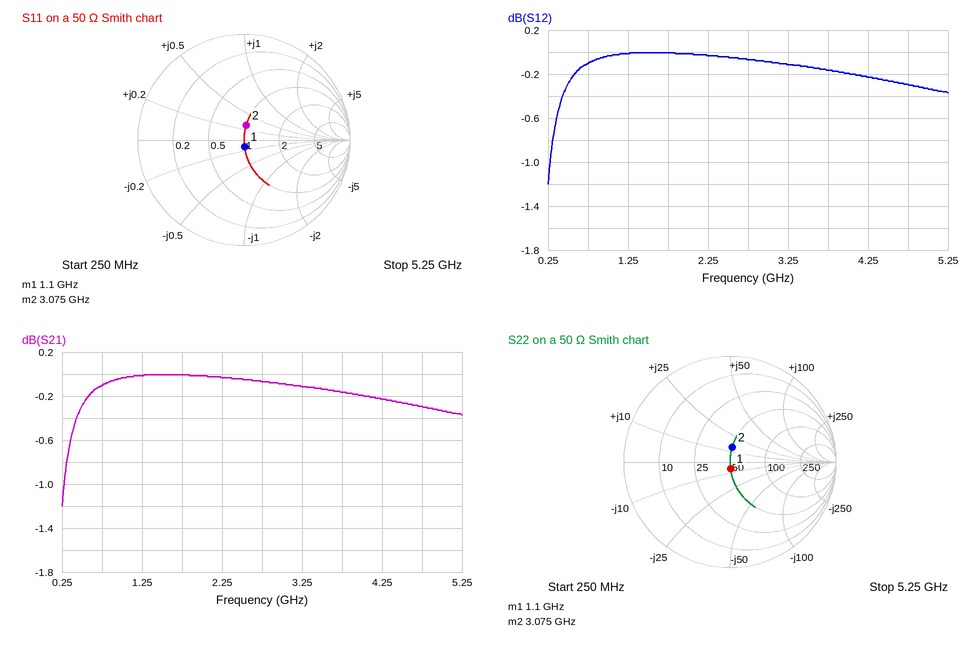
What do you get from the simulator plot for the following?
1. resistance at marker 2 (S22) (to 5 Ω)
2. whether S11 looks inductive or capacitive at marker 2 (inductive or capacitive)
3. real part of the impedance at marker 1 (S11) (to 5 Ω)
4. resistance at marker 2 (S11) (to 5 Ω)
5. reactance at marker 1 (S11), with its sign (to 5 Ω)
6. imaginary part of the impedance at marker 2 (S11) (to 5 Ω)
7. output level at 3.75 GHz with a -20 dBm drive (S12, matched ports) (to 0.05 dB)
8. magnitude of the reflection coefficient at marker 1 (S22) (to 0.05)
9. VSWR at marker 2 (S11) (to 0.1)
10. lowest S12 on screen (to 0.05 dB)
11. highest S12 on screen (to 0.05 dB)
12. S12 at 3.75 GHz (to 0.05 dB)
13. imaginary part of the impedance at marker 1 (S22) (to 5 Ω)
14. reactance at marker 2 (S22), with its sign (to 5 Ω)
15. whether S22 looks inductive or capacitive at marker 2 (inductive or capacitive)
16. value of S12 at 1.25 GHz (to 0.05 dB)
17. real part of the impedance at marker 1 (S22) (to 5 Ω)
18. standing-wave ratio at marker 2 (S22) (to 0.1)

50 Ω
inductive
50 Ω
50 Ω
-5 Ω
+15 Ω
-20.15 dBm
0.05
1.3
-1.20 dB
0.00 dB
-0.15 dB
-5 Ω
+15 Ω
inductive
0.00 dB
50 Ω
1.3
